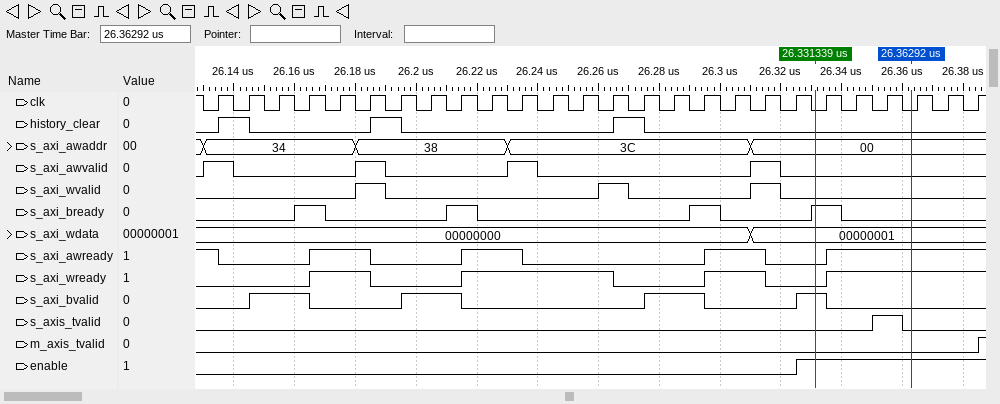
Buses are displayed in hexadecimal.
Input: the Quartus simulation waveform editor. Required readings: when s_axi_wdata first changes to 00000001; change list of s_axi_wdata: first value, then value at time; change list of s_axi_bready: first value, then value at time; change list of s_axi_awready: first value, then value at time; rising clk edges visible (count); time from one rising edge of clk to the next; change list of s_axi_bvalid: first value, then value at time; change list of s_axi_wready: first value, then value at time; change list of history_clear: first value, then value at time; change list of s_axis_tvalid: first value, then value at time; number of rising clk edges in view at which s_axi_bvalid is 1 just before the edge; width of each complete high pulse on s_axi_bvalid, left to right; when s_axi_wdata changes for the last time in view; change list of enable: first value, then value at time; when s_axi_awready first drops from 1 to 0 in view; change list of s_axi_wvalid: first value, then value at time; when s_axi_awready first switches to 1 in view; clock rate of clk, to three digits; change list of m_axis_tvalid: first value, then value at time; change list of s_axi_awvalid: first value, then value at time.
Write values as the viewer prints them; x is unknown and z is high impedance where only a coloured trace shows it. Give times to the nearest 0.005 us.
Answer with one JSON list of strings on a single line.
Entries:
["26.31 us", "00000000, 00000001 at 26.31 us", "0, 1 at 26.16 us, 0 at 26.17 us, 1 at 26.21 us, 0 at 26.22 us, 1 at 26.29 us, 0 at 26.3 us, 1 at 26.33 us, 0 at 26.34 us", "1, 0 at 26.135 us, 1 at 26.165 us, 0 at 26.185 us, 1 at 26.215 us, 0 at 26.235 us, 1 at 26.295 us, 0 at 26.315 us, 1 at 26.335 us", "26", "0.01 us", "0, 1 at 26.145 us, 0 at 26.165 us, 1 at 26.195 us, 0 at 26.215 us, 1 at 26.275 us, 0 at 26.295 us, 1 at 26.325 us, 0 at 26.335 us", "0, 1 at 26.165 us, 0 at 26.185 us, 1 at 26.215 us, 0 at 26.265 us, 1 at 26.295 us, 0 at 26.315 us, 1 at 26.335 us", "0, 1 at 26.135 us, 0 at 26.145 us, 1 at 26.185 us, 0 at 26.195 us, 1 at 26.265 us, 0 at 26.275 us", "0, 1 at 26.35 us, 0 at 26.36 us", "7", "0.02 us, 0.02 us, 0.02 us, 0.01 us", "26.31 us", "0, 1 at 26.325 us", "26.135 us", "0, 1 at 26.18 us, 0 at 26.19 us, 1 at 26.26 us, 0 at 26.27 us, 1 at 26.31 us, 0 at 26.32 us", "26.165 us", "100 MHz", "0, 1 at 26.385 us", "0, 1 at 26.13 us, 0 at 26.14 us, 1 at 26.18 us, 0 at 26.19 us, 1 at 26.23 us, 0 at 26.24 us, 1 at 26.31 us, 0 at 26.32 us"]
